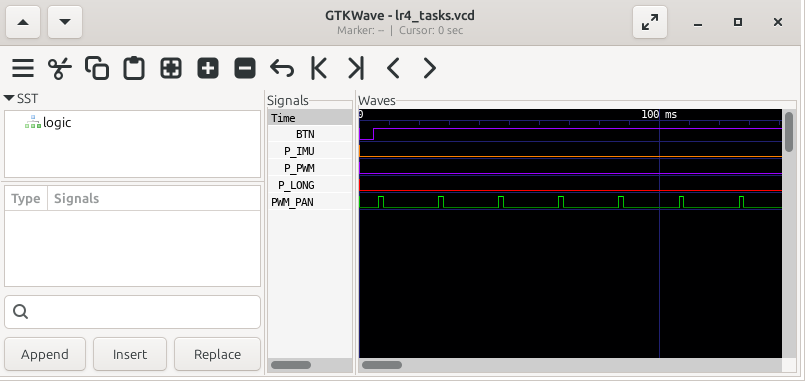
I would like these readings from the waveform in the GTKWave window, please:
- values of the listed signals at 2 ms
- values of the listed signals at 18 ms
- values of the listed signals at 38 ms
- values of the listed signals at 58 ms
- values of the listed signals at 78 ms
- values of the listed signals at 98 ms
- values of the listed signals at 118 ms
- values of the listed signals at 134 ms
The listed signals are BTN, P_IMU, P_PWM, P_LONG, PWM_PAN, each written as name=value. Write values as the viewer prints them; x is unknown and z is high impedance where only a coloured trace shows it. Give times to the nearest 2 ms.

BTN=0, P_IMU=0, P_PWM=0, P_LONG=0, PWM_PAN=0
BTN=1, P_IMU=0, P_PWM=0, P_LONG=0, PWM_PAN=0
BTN=1, P_IMU=0, P_PWM=0, P_LONG=0, PWM_PAN=0
BTN=1, P_IMU=0, P_PWM=0, P_LONG=0, PWM_PAN=0
BTN=1, P_IMU=0, P_PWM=0, P_LONG=0, PWM_PAN=0
BTN=1, P_IMU=0, P_PWM=0, P_LONG=0, PWM_PAN=0
BTN=1, P_IMU=0, P_PWM=0, P_LONG=0, PWM_PAN=0
BTN=1, P_IMU=0, P_PWM=0, P_LONG=0, PWM_PAN=0
